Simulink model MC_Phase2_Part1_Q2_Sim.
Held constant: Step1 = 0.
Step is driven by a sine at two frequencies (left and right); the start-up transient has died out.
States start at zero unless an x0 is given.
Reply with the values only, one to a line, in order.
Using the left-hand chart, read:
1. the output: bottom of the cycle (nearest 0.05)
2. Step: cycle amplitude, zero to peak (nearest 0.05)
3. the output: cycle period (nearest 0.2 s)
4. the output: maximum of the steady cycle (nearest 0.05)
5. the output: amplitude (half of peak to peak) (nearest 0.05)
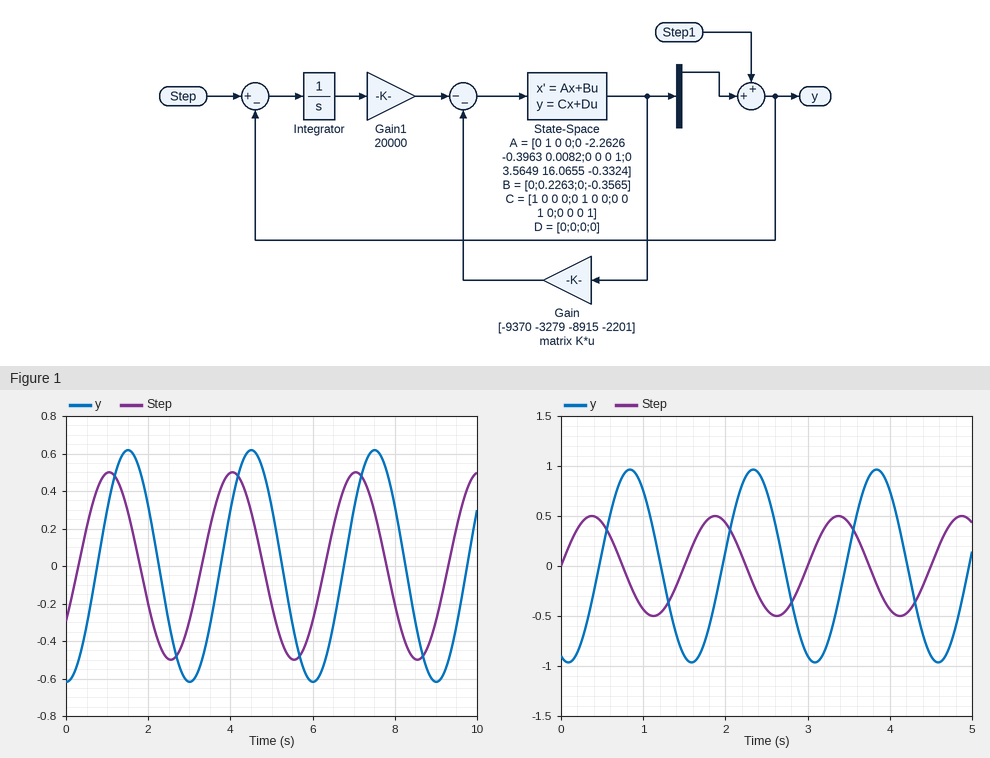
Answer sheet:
-0.60
0.50
3.0 s
0.60
0.60
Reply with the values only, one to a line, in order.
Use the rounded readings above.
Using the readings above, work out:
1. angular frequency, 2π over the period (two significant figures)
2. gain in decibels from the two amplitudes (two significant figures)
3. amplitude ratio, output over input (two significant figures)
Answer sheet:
2.1 rad/s
1.6 dB
1.2
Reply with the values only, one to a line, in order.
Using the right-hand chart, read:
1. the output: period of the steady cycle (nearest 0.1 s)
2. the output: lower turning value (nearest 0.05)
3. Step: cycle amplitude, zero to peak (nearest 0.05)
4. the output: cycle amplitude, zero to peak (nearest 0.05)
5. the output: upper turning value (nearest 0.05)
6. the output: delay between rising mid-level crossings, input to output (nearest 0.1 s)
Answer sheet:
1.5 s
-0.95
0.50
0.95
0.95
0.5 s
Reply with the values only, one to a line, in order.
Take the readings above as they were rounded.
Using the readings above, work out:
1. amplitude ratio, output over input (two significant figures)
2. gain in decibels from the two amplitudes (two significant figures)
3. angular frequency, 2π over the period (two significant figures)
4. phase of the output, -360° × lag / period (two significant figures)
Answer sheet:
1.9
5.6 dB
4.2 rad/s
-120°
